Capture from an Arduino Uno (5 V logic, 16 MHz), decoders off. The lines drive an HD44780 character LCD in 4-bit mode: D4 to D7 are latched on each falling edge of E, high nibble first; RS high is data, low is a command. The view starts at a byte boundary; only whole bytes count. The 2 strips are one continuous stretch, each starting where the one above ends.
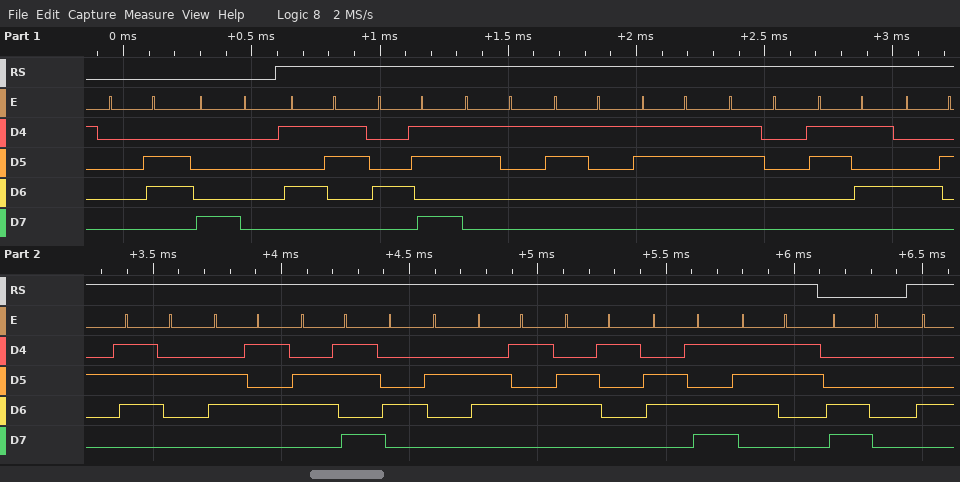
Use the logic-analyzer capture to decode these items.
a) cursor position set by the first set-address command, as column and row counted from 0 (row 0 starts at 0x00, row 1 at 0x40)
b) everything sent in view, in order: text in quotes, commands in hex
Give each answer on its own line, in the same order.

column 0, row 0
0x06 0x80 "SK11305BrekBeams" 0xC0
